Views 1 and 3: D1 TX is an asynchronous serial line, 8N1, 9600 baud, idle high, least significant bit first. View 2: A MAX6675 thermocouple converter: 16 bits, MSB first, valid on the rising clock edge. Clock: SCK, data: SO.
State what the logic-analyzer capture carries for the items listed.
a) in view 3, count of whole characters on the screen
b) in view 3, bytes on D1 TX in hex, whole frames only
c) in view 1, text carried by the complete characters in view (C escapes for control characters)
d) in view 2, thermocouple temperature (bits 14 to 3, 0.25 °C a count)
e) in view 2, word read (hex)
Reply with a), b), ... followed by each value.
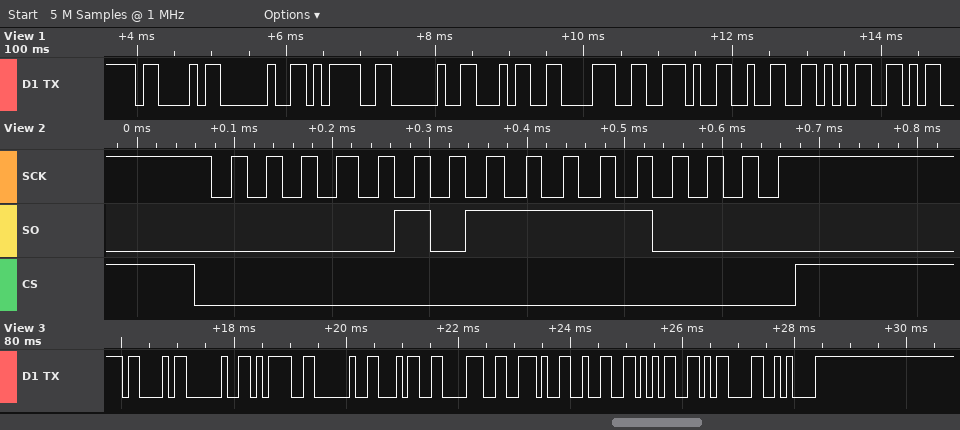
a) 11
b) 43 20 3D 20 34 38 2E 32 35 0D 0A
c) "C = 48.25"
d) 47.50 °C
e) 0x05F0
